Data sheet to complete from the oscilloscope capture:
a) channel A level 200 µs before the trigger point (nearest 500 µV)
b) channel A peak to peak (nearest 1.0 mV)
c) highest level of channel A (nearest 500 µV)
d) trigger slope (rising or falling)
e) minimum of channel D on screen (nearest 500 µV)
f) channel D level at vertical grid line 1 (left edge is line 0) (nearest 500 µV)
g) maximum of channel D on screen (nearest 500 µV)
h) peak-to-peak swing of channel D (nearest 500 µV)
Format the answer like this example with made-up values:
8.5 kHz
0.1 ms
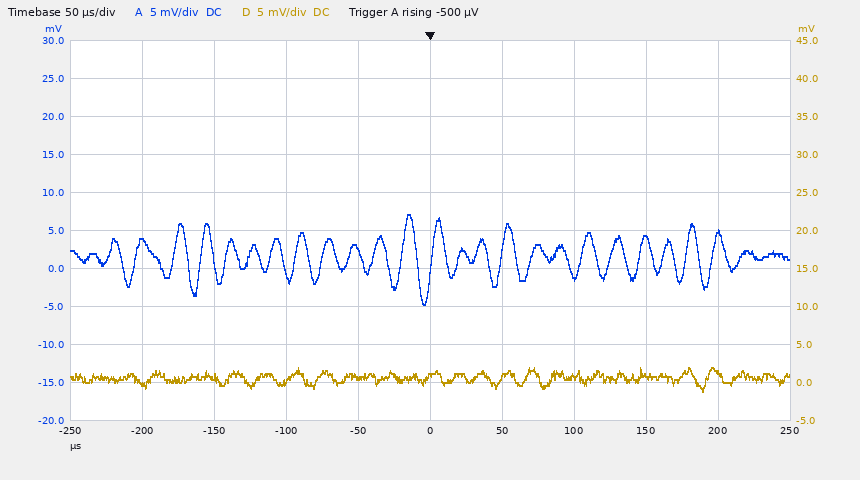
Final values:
3.5 mV
12.0 mV
7.0 mV
rising
-1.0 mV
0.0 mV
2.0 mV
3.0 mV
